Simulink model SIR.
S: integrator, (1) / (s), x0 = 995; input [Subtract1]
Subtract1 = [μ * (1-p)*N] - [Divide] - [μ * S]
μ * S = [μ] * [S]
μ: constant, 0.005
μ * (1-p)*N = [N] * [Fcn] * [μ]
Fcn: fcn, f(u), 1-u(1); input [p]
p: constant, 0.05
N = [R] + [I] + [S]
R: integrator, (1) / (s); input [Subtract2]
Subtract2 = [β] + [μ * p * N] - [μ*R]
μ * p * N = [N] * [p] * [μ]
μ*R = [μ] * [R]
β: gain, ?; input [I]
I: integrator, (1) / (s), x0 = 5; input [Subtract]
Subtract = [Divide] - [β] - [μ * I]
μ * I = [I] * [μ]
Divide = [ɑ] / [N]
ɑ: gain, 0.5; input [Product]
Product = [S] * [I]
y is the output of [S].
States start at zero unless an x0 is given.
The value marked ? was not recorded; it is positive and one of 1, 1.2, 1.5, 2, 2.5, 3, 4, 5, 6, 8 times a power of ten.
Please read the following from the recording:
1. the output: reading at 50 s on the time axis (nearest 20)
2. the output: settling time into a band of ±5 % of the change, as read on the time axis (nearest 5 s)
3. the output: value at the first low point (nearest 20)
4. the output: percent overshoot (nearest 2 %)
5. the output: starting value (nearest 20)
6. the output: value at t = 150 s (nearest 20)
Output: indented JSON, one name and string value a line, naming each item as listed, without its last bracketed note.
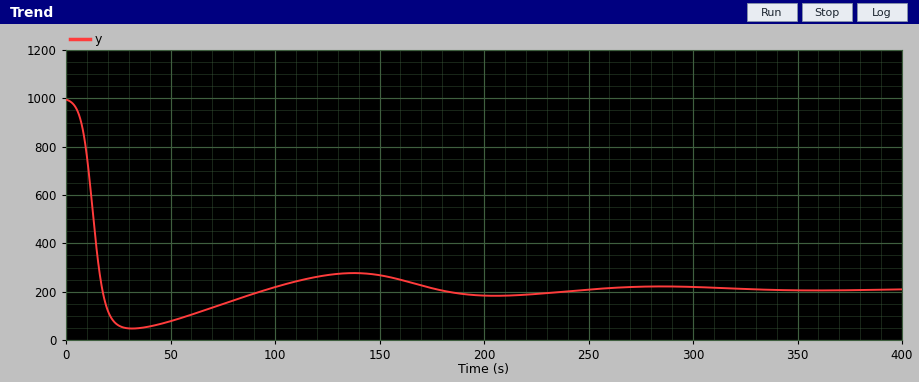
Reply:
{
  "the output: reading at 50 s on the time axis": "80",
  "the output: settling time into a band of ±5 % of the change, as read on the time axis": "160 s",
  "the output: value at the first low point": "40",
  "the output: percent overshoot": "20 %",
  "the output: starting value": "1000",
  "the output: value at t = 150 s": "260"
}
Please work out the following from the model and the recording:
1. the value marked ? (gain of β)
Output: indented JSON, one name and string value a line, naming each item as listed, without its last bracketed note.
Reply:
{
  "the value marked ?": "0.1"
}
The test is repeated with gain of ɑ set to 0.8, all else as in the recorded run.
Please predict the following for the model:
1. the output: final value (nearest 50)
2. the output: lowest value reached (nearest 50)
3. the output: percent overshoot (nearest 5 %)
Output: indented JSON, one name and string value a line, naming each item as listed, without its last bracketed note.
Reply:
{
  "the output: final value": "150",
  "the output: lowest value reached": "0",
  "the output: percent overshoot": "15 %"
}
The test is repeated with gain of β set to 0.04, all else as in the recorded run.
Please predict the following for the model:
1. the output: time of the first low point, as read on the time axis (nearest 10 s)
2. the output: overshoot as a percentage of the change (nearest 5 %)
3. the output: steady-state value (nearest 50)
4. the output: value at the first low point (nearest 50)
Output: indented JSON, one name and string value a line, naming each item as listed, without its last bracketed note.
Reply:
{
  "the output: time of the first low point, as read on the time axis": "30 s",
  "the output: overshoot as a percentage of the change": "10 %",
  "the output: steady-state value": "100",
  "the output: value at the first low point": "0"
}
